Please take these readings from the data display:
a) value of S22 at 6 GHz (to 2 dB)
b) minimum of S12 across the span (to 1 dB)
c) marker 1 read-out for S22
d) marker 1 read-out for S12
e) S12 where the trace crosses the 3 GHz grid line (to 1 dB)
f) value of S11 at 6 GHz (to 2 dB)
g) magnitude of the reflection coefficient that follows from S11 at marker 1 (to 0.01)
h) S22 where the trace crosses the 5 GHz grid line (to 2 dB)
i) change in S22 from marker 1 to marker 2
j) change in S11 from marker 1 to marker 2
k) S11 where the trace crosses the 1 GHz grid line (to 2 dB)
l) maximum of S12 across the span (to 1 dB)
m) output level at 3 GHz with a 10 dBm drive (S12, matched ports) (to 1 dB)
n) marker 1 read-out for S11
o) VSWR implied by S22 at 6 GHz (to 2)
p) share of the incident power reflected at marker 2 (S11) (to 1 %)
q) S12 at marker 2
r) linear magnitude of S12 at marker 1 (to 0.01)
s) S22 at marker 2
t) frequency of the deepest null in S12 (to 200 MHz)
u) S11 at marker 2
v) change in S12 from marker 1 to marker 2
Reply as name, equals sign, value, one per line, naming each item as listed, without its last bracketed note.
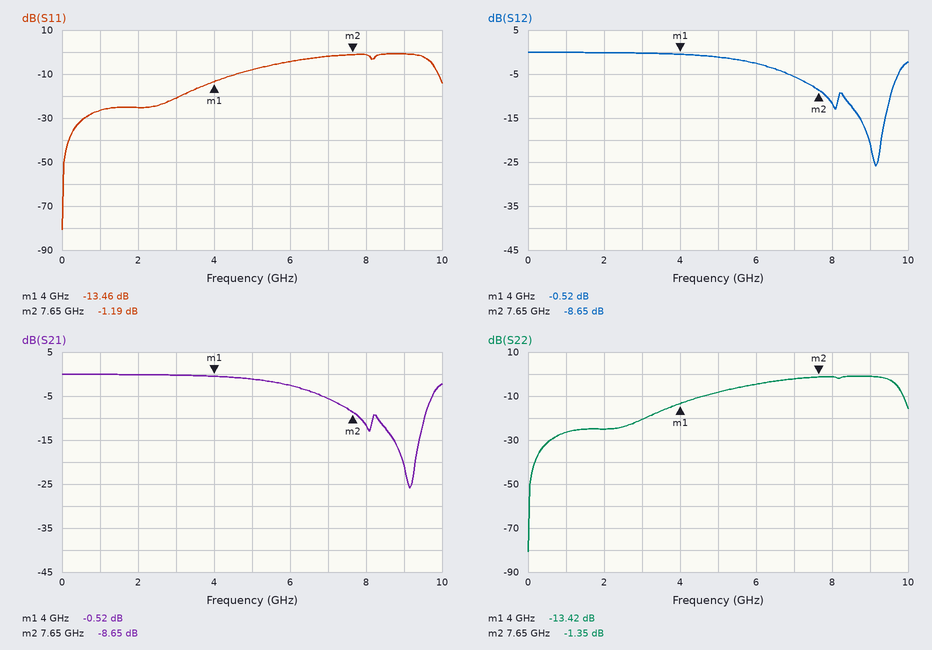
value of S22 at 6 GHz = -4 dB
minimum of S12 across the span = -26 dB
marker 1 read-out for S22 = -13.42 dB
marker 1 read-out for S12 = -0.52 dB
S12 where the trace crosses the 3 GHz grid line = 0 dB
value of S11 at 6 GHz = -4 dB
magnitude of the reflection coefficient that follows from S11 at marker 1 = 0.21
S22 where the trace crosses the 5 GHz grid line = -8 dB
change in S22 from marker 1 to marker 2 = 12.07 dB
change in S11 from marker 1 to marker 2 = 12.27 dB
S11 where the trace crosses the 1 GHz grid line = -26 dB
maximum of S12 across the span = 0 dB
output level at 3 GHz with a 10 dBm drive (S12, matched ports) = 10 dBm
marker 1 read-out for S11 = -13.46 dB
VSWR implied by S22 at 6 GHz = 4
share of the incident power reflected at marker 2 (S11) = 76 %
S12 at marker 2 = -8.65 dB
linear magnitude of S12 at marker 1 = 0.94
S22 at marker 2 = -1.35 dB
frequency of the deepest null in S12 = 9.2 GHz
S11 at marker 2 = -1.19 dB
change in S12 from marker 1 to marker 2 = -8.13 dB
